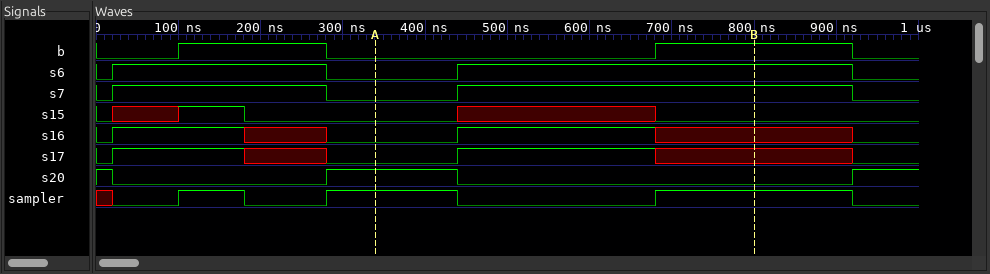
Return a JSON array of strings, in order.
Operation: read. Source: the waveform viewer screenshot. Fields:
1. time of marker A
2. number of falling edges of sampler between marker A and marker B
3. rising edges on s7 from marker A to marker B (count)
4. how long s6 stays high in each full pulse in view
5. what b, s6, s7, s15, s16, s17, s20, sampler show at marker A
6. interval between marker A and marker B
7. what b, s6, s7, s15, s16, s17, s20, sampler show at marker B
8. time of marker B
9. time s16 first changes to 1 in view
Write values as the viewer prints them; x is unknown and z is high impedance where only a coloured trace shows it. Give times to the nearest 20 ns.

["340 ns", "1", "1", "260 ns, 480 ns", "b=0, s6=0, s7=0, s15=0, s16=0, s17=0, s20=1, sampler=1", "460 ns", "b=1, s6=1, s7=1, s15=0, s16=x, s17=x, s20=0, sampler=1", "800 ns", "20 ns"]
